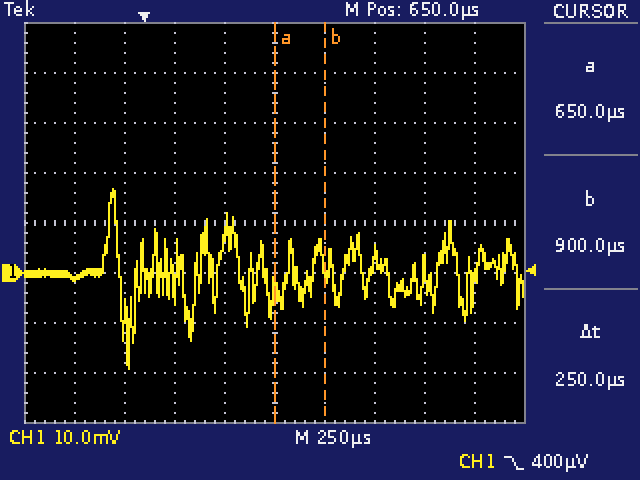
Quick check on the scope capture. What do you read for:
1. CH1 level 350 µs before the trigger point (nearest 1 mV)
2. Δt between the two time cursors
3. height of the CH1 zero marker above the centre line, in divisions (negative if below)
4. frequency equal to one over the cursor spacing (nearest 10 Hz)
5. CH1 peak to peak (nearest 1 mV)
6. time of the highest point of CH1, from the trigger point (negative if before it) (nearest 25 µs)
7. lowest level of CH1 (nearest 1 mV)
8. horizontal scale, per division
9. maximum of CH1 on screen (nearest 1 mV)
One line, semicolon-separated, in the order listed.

-1 mV; 250 µs; -1.0 div; 4.00 kHz; 36 mV; -150 µs; -19 mV; 250 µs; 17 mV
